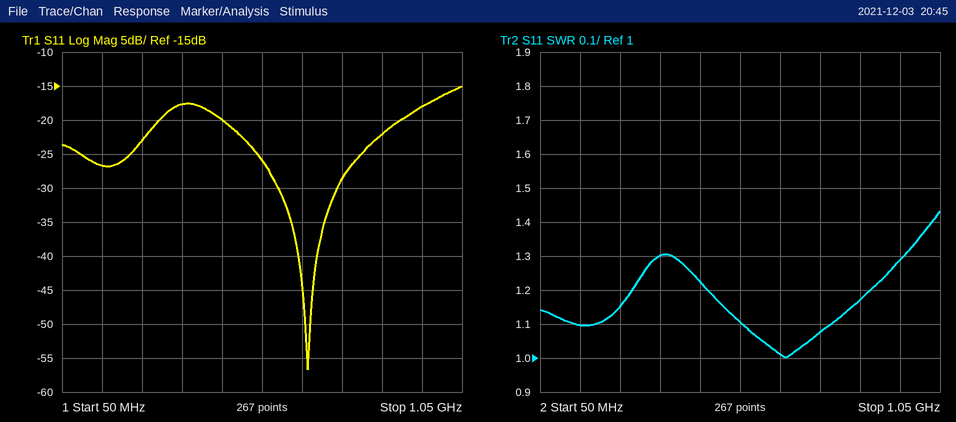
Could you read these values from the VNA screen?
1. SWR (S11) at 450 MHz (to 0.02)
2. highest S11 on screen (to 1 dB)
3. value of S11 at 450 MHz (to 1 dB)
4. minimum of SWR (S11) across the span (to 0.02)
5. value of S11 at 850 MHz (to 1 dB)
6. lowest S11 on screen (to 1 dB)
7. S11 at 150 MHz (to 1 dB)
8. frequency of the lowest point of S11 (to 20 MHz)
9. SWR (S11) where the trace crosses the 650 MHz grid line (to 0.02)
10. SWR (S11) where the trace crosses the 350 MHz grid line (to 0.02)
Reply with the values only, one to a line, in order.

1.22
-15 dB
-20 dB
1.00
-22 dB
-57 dB
-27 dB
660 MHz
1.02
1.30
